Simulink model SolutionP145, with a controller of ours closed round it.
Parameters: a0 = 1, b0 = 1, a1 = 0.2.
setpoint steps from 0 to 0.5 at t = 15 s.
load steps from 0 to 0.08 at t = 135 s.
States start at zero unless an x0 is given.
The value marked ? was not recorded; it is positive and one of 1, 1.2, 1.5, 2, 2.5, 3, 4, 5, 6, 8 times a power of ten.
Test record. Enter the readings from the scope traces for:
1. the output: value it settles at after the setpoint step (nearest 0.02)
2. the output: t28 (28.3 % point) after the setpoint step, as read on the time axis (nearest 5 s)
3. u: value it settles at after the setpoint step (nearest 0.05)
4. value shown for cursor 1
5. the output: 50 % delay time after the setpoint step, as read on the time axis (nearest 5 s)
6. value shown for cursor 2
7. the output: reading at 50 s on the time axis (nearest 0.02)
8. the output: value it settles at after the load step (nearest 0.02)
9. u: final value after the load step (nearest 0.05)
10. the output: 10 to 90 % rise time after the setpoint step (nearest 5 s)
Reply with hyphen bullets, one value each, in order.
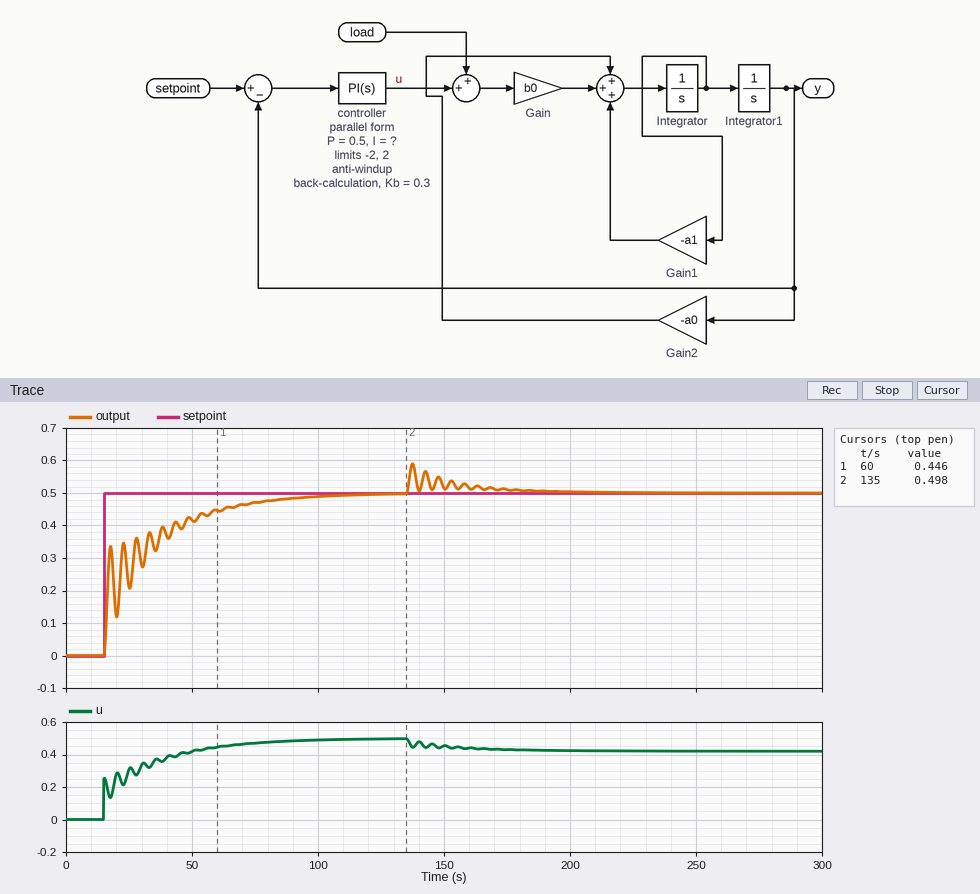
- 0.50
- 15 s
- 0.50
- 0.446
- 15 s
- 0.498
- 0.42
- 0.50
- 0.40
- 45 s
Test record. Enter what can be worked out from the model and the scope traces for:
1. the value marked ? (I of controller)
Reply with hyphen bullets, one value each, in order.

- 0.06
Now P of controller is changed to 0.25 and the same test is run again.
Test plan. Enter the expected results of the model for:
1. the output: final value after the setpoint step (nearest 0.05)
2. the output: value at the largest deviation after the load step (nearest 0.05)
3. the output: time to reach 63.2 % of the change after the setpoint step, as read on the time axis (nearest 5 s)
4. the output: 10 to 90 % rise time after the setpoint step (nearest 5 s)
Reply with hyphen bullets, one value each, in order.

- 0.50
- 0.60
- 30 s
- 40 s
